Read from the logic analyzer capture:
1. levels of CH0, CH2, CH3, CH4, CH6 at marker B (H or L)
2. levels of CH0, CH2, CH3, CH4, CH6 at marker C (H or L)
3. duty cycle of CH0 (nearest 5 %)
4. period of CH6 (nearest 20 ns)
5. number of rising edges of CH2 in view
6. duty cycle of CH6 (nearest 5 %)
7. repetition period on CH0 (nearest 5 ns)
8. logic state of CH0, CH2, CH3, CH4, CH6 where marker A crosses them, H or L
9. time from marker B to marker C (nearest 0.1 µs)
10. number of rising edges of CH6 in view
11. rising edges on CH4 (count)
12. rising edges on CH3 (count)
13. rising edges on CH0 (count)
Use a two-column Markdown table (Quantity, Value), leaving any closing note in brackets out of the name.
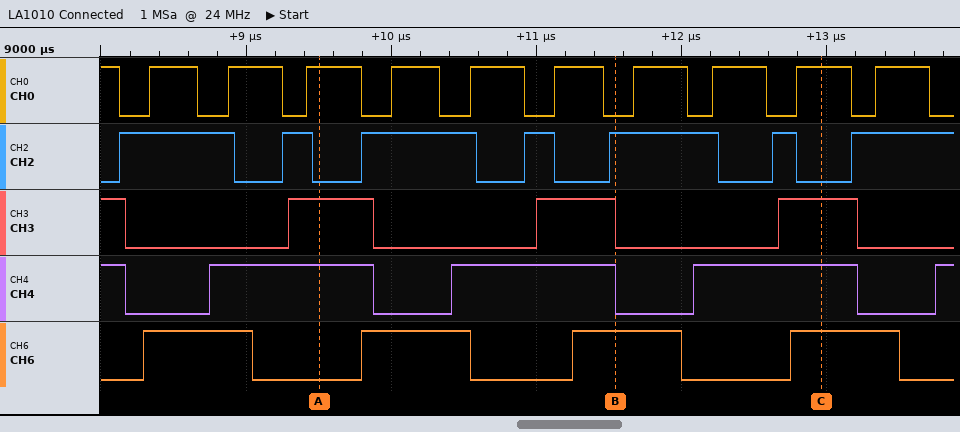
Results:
| Quantity | Value |
|---|---|
| levels of CH0, CH2, CH3, CH4, CH6 at marker B | CH0=L, CH2=H, CH3=L, CH4=L, CH6=H |
| levels of CH0, CH2, CH3, CH4, CH6 at marker C | CH0=H, CH2=L, CH3=H, CH4=H, CH6=H |
| duty cycle of CH0 | 65 % |
| period of CH6 | 1480 ns |
| number of rising edges of CH2 in view | 7 |
| duty cycle of CH6 | 50 % |
| repetition period on CH0 | 555 ns |
| logic state of CH0, CH2, CH3, CH4, CH6 where marker A crosses them, H or L | CH0=H, CH2=L, CH3=H, CH4=H, CH6=L |
| time from marker B to marker C | 1.4 µs |
| number of rising edges of CH6 in view | 4 |
| rising edges on CH4 | 4 |
| rising edges on CH3 | 3 |
| rising edges on CH0 | 10 |
